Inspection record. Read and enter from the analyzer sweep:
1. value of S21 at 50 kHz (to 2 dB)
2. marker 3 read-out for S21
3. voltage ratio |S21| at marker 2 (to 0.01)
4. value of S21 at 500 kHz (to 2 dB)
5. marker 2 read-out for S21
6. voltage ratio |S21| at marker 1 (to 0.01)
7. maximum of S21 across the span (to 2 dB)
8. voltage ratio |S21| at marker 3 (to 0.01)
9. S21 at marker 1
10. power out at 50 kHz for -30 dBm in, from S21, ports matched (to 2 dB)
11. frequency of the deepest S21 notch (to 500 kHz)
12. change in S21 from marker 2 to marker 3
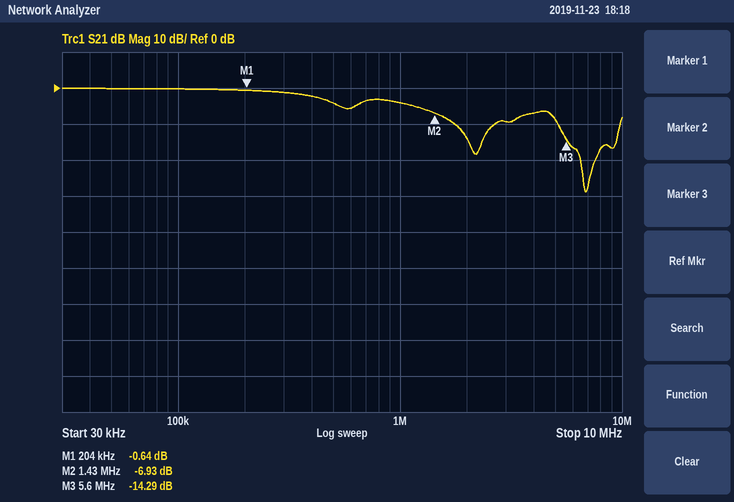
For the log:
0 dB
-14.29 dB
0.45
-4 dB
-6.93 dB
0.93
0 dB
0.19
-0.64 dB
-30 dBm
7.0 MHz
-7.36 dB
